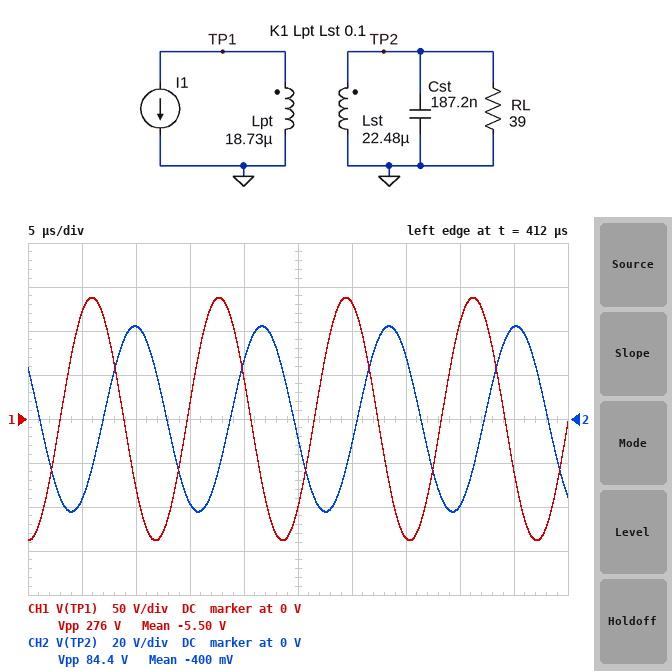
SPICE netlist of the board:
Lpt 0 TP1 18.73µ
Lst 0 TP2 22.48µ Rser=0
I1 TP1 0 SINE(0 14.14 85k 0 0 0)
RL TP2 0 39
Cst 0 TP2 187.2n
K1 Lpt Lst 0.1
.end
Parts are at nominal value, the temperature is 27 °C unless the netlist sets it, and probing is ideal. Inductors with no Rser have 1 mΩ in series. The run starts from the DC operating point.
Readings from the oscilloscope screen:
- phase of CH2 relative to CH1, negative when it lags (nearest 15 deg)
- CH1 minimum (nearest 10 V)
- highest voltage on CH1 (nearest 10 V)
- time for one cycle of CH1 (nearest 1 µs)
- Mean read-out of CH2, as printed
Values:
-120 deg
-140 V
140 V
12 µs
-400 mV
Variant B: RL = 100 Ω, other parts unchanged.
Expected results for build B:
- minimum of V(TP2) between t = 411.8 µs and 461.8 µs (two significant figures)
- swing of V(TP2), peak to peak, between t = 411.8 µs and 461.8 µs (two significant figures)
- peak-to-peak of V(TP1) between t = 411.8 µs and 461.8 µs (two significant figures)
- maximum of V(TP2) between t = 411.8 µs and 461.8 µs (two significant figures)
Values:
-66 V
130 V
270 V
66 V
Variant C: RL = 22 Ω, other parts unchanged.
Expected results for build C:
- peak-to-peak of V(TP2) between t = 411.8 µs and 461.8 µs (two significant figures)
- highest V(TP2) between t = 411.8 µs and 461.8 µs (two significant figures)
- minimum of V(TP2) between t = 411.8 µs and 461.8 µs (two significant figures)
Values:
53 V
27 V
-27 V
